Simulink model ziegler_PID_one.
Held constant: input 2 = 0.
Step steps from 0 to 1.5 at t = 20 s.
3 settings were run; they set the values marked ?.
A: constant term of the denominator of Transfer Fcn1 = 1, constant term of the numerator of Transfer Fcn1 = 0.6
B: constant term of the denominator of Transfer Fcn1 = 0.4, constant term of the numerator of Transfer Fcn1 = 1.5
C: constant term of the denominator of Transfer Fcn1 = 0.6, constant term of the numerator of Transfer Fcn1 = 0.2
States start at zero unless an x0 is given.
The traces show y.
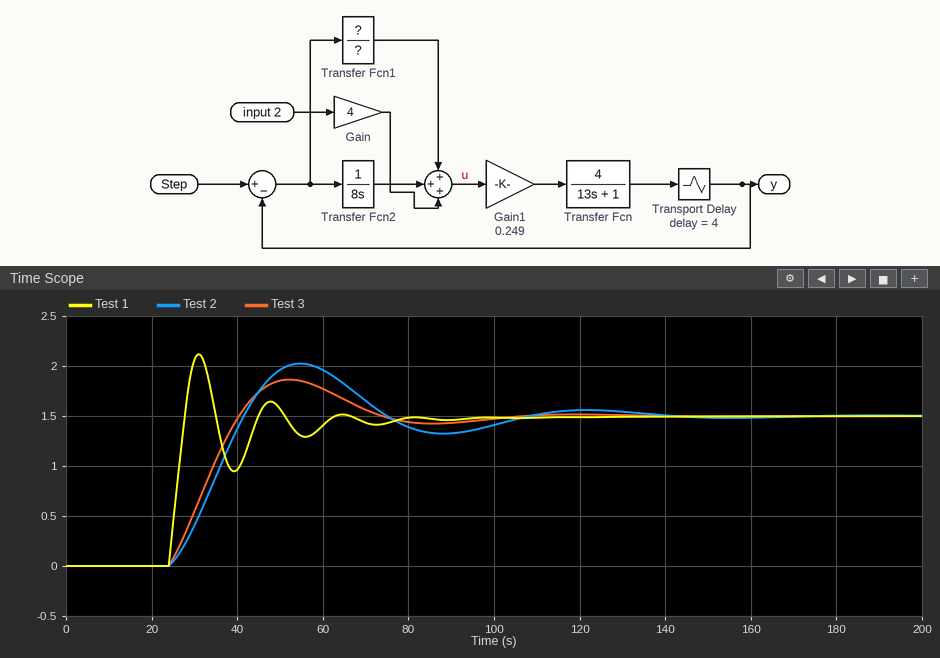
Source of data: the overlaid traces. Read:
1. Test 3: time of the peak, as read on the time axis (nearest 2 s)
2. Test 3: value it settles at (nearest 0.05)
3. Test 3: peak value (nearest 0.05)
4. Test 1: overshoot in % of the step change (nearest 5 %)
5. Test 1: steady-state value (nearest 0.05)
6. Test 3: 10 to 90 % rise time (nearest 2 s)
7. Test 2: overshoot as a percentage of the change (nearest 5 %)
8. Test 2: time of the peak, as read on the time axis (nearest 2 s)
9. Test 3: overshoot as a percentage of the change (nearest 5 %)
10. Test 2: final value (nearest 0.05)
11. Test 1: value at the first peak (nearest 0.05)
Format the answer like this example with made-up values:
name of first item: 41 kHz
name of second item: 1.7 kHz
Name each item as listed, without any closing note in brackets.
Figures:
Test 3: time of the peak, as read on the time axis: 52 s
Test 3: value it settles at: 1.50
Test 3: peak value: 1.85
Test 1: overshoot in % of the step change: 40 %
Test 1: steady-state value: 1.50
Test 3: 10 to 90 % rise time: 12 s
Test 2: overshoot as a percentage of the change: 35 %
Test 2: time of the peak, as read on the time axis: 54 s
Test 3: overshoot as a percentage of the change: 25 %
Test 2: final value: 1.50
Test 1: value at the first peak: 2.10
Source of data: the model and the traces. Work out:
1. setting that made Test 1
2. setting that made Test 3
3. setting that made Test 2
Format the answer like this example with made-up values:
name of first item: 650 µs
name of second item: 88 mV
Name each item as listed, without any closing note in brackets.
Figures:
setting that made Test 1: B
setting that made Test 3: A
setting that made Test 2: C
